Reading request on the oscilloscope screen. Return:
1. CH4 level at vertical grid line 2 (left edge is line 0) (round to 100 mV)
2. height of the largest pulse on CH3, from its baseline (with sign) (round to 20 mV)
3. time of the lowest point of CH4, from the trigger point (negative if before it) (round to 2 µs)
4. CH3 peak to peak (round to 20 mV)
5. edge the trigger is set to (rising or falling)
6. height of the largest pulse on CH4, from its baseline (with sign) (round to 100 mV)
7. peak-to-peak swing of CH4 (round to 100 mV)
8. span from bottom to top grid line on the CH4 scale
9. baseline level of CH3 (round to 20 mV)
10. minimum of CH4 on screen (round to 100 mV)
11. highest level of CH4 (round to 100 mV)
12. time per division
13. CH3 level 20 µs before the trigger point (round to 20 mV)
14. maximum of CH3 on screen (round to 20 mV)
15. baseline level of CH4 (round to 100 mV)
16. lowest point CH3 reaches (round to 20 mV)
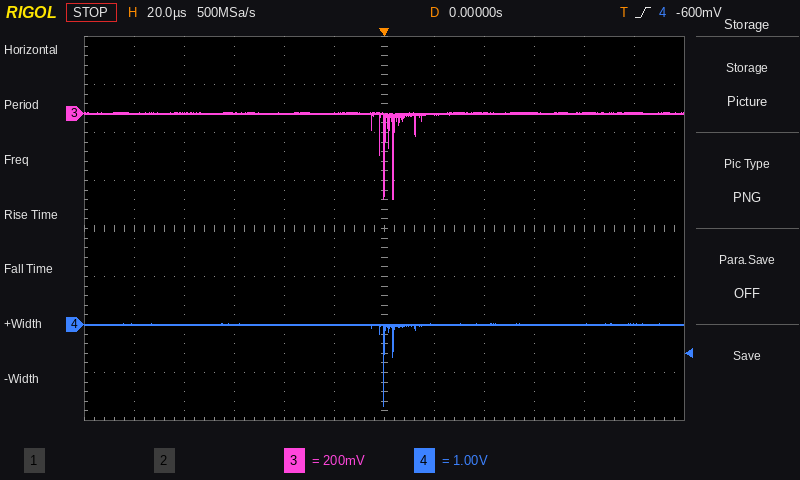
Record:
0.0 V
-360 mV
0 µs
360 mV
rising
-1.7 V
1.7 V
8 V
0 mV
-1.7 V
0.0 V
20 µs
0 mV
0 mV
0.0 V
-360 mV
